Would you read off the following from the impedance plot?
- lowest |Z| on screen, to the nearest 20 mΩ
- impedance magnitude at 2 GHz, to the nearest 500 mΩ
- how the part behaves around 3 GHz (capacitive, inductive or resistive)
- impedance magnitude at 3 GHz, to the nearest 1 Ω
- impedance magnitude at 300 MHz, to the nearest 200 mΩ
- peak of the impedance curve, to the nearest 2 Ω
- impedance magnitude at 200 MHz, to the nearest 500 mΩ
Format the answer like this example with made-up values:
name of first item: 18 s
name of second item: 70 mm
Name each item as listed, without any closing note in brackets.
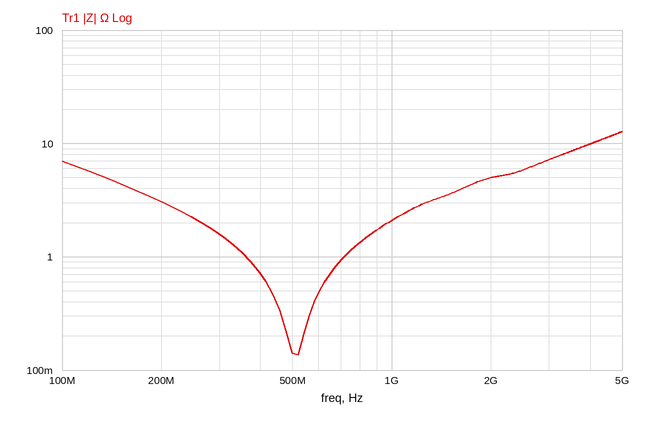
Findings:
lowest |Z| on screen, to the nearest 20 mΩ: 140 mΩ
impedance magnitude at 2 GHz, to the nearest 500 mΩ: 5.0 Ω
how the part behaves around 3 GHz: inductive
impedance magnitude at 3 GHz, to the nearest 1 Ω: 7 Ω
impedance magnitude at 300 MHz, to the nearest 200 mΩ: 1.6 Ω
peak of the impedance curve, to the nearest 2 Ω: 12 Ω
impedance magnitude at 200 MHz, to the nearest 500 mΩ: 3.0 Ω
